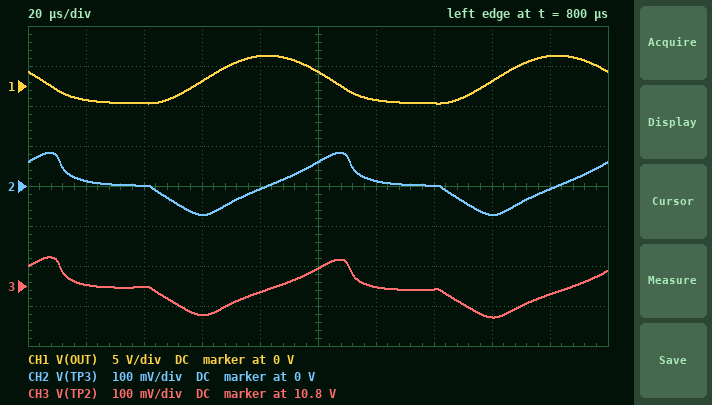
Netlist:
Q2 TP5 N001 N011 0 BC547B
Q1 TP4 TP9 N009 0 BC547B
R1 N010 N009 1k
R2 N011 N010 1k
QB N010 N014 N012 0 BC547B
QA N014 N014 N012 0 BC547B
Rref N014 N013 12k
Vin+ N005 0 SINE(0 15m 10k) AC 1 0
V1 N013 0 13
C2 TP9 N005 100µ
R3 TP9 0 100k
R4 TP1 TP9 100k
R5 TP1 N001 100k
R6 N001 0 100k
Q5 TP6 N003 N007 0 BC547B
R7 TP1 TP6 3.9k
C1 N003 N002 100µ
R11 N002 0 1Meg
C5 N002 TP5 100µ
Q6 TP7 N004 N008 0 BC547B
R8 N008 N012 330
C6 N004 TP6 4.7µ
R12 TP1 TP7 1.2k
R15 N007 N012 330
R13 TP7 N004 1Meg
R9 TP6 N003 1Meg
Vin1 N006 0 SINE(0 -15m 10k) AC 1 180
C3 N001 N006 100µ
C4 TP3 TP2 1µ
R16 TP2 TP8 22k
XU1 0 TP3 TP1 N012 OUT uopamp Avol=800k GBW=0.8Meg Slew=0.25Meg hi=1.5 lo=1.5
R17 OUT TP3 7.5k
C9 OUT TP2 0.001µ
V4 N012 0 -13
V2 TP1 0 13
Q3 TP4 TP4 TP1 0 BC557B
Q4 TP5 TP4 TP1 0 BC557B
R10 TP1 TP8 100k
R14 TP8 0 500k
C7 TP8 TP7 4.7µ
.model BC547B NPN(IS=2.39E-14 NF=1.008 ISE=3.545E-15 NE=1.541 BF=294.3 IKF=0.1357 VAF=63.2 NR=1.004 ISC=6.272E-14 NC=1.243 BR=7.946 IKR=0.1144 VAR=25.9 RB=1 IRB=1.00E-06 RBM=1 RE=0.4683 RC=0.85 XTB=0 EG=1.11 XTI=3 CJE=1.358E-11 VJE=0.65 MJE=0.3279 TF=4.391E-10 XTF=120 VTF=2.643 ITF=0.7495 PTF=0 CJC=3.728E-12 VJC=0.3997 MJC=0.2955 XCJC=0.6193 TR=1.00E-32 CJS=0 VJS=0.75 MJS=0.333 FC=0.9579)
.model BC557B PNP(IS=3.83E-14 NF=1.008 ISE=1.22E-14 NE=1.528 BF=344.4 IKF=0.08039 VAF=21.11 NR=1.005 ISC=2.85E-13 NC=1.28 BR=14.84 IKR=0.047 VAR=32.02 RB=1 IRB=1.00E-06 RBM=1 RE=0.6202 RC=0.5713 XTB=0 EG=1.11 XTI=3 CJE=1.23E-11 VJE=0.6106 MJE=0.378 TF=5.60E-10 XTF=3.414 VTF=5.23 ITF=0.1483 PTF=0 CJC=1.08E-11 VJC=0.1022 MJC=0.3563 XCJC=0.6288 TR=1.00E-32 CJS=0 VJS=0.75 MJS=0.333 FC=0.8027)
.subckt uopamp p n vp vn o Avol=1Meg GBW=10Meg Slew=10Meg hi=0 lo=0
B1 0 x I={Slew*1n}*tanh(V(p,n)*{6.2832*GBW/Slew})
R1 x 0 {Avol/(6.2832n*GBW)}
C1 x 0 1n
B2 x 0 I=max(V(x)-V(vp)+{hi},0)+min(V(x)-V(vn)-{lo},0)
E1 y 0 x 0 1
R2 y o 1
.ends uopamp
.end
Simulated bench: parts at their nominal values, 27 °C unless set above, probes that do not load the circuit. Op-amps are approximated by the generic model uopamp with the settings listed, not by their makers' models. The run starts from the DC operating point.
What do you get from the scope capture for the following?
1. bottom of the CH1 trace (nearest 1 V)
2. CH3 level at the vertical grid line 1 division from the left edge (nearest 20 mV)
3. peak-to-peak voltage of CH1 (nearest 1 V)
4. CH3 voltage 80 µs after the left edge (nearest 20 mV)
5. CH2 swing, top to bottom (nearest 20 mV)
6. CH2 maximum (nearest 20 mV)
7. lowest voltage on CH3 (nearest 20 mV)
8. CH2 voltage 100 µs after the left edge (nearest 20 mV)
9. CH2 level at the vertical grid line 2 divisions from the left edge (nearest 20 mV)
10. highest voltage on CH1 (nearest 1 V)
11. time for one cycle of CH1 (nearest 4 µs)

-2 V
10.80 V
6 V
10.78 V
160 mV
80 mV
10.72 V
60 mV
0 V
4 V
100 µs
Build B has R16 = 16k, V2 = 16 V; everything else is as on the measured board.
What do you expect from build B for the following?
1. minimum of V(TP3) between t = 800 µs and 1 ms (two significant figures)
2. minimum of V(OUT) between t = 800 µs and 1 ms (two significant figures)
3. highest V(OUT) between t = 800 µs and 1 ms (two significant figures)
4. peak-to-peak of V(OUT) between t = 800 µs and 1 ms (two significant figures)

-590 mV
-3.3 V
5.0 V
8.3 V
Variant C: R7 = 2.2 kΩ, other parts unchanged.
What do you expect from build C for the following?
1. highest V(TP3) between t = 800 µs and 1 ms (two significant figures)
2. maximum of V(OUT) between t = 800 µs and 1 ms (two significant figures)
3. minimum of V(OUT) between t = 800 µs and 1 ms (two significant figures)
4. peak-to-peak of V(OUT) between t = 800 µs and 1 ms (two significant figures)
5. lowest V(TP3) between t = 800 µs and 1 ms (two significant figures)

33 mV
2.4 V
-2.1 V
4.5 V
-34 mV
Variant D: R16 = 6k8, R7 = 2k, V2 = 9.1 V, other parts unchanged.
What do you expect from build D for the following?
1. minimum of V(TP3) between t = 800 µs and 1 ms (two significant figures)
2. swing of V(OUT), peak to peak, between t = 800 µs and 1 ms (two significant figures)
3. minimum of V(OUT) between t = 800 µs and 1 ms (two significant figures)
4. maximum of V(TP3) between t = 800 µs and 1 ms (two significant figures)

-1.5 V
11 V
-5.0 V
1.3 V
